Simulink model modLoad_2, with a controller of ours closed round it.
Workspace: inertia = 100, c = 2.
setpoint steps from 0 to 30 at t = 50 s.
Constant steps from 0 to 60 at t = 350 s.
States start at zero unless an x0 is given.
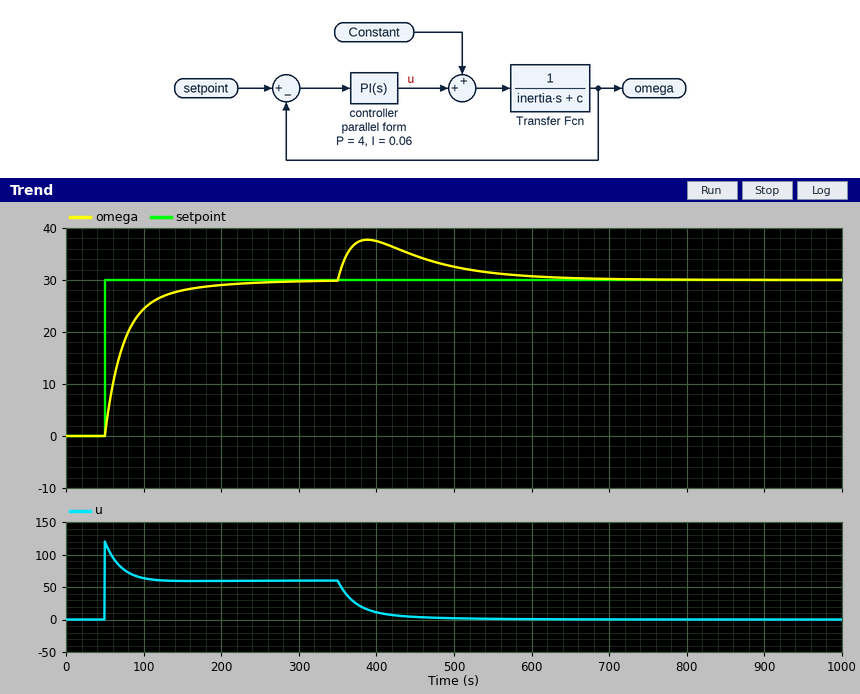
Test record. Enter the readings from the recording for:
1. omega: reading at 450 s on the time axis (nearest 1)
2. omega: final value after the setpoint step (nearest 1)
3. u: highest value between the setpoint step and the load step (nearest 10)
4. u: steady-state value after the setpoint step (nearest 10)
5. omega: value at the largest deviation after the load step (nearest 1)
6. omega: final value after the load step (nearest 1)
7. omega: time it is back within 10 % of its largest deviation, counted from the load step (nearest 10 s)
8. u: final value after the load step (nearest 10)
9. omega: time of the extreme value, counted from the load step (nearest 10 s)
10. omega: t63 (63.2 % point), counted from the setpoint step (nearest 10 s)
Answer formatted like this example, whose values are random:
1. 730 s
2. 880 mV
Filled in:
1. 35
2. 30
3. 120
4. 60
5. 38
6. 30
7. 240 s
8. 0
9. 40 s
10. 30 s
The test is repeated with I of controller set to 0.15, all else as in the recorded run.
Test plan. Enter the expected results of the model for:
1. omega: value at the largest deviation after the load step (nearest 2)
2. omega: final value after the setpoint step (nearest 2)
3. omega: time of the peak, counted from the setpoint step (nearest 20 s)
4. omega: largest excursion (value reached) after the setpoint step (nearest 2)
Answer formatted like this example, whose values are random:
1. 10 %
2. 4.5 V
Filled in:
1. 36
2. 30
3. 80 s
4. 32
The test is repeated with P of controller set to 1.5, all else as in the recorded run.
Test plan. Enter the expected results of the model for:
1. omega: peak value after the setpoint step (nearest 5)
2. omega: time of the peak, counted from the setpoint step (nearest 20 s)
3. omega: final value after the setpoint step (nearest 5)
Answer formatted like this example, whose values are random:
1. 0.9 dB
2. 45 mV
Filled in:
1. 30
2. 140 s
3. 30
